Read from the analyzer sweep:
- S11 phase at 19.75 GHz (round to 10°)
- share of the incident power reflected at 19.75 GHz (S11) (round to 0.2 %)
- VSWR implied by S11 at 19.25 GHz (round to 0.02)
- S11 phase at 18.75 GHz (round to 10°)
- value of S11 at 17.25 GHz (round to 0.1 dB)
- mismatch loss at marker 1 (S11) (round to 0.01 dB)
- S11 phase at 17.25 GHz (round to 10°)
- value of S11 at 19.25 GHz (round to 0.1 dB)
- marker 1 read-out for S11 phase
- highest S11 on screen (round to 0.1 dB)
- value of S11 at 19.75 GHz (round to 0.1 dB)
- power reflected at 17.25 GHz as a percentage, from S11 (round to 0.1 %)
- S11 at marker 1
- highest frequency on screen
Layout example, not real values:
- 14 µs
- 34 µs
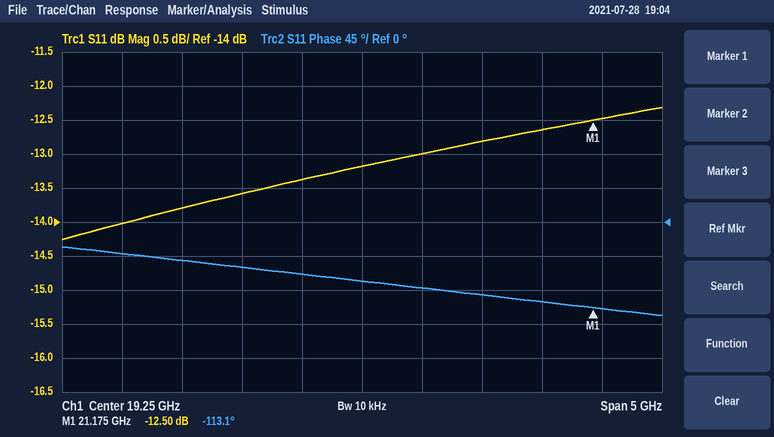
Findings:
- -90°
- 5.0 %
- 1.56
- -70°
- -14.0 dB
- 0.25 dB
- -40°
- -13.2 dB
- -113.1°
- -12.3 dB
- -13.0 dB
- 4.0 %
- -12.50 dB
- 21.75 GHz
